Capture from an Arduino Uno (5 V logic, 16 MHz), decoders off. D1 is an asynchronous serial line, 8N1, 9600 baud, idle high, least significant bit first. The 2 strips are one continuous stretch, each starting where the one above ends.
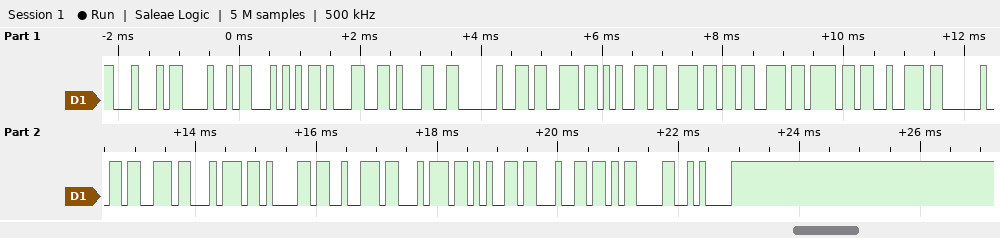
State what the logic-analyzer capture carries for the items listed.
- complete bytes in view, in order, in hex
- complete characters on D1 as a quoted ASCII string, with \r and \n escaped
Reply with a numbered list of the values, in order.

1. 44 48 54 31 31 20 73 65 6E 73 6F 72 20 73 74 61 72 74 65 64 0D 0A
2. "DHT11 sensor started\r\n"
